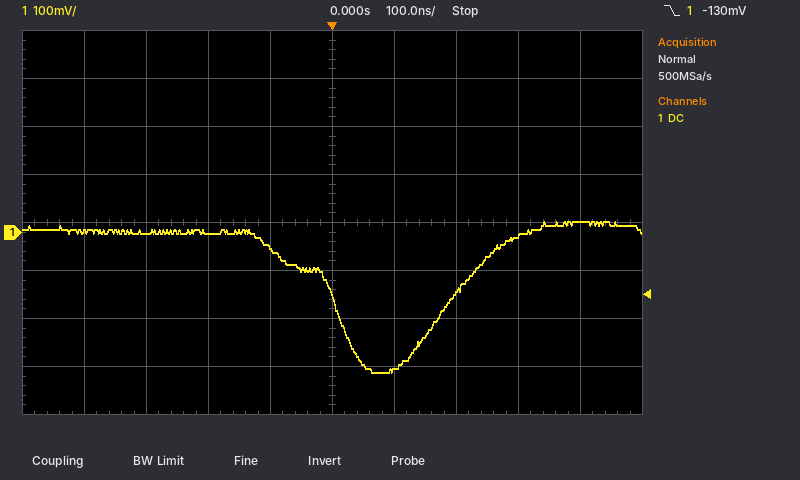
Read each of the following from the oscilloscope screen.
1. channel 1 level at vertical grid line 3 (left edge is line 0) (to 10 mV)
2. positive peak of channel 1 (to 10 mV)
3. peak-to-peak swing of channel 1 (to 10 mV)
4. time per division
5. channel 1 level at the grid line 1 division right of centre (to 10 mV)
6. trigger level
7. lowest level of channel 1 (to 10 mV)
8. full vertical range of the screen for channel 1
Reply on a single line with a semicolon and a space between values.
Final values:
0 mV; 20 mV; 310 mV; 100 ns; -290 mV; -130 mV; -290 mV; 800 mV
